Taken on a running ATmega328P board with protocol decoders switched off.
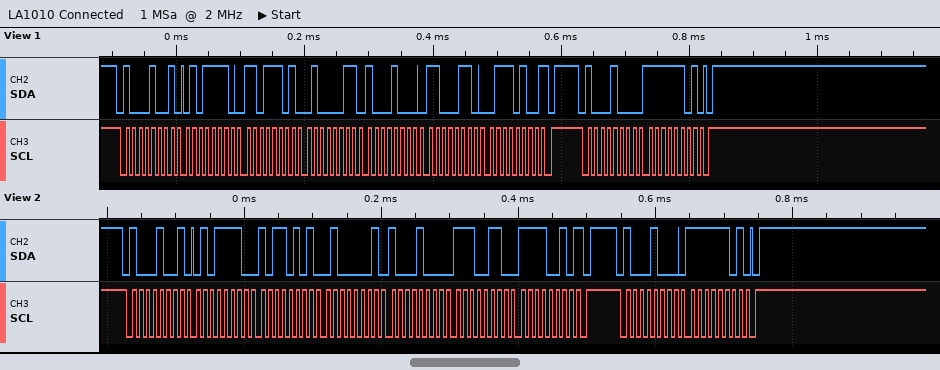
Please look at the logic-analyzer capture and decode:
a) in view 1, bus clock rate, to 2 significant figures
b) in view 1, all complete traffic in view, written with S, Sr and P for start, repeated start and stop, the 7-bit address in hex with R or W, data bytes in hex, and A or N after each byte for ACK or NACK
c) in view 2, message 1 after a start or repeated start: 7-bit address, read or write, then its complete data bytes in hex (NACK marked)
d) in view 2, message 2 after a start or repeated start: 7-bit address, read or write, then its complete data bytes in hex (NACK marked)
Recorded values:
100 kHz
S 44R A 5E A DD A 43 A 88 A C6 A 74 N P S 44W A FD A P
0x44 read: 5E B5 41 88 E6 F2 NACK
0x44 write: FD
